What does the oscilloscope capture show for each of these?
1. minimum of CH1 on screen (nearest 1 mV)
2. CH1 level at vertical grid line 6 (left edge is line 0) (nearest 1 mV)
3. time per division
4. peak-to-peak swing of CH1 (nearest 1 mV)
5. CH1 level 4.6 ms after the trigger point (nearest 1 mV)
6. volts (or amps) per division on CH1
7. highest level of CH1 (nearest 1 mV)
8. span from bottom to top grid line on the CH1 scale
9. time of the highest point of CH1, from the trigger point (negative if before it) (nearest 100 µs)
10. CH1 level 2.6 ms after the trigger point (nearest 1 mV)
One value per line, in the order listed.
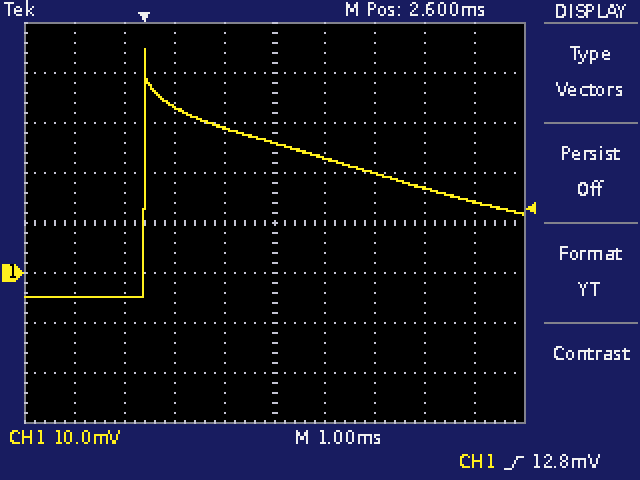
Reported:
-5 mV
23 mV
1 ms
50 mV
20 mV
10 mV
45 mV
80 mV
0.0 ms
26 mV
